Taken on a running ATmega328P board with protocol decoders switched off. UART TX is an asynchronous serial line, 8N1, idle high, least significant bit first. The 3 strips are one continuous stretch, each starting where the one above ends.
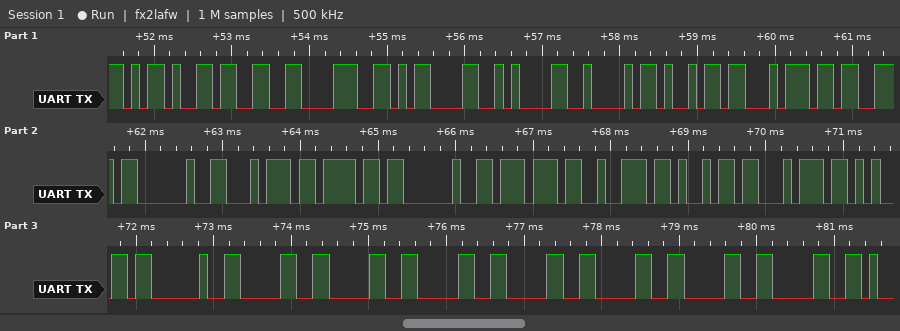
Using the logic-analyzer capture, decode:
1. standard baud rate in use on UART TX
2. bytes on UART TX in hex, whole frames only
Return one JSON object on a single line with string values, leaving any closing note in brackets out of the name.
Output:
{"standard baud rate in use on UART TX": "9600 baud", "bytes on UART TX in hex, whole frames only": "2D 33 38 0D 0A 42 69 74 73 20 74 6F 20 77 72 69 74 65 20 30 30 30 30 30 30 30"}
